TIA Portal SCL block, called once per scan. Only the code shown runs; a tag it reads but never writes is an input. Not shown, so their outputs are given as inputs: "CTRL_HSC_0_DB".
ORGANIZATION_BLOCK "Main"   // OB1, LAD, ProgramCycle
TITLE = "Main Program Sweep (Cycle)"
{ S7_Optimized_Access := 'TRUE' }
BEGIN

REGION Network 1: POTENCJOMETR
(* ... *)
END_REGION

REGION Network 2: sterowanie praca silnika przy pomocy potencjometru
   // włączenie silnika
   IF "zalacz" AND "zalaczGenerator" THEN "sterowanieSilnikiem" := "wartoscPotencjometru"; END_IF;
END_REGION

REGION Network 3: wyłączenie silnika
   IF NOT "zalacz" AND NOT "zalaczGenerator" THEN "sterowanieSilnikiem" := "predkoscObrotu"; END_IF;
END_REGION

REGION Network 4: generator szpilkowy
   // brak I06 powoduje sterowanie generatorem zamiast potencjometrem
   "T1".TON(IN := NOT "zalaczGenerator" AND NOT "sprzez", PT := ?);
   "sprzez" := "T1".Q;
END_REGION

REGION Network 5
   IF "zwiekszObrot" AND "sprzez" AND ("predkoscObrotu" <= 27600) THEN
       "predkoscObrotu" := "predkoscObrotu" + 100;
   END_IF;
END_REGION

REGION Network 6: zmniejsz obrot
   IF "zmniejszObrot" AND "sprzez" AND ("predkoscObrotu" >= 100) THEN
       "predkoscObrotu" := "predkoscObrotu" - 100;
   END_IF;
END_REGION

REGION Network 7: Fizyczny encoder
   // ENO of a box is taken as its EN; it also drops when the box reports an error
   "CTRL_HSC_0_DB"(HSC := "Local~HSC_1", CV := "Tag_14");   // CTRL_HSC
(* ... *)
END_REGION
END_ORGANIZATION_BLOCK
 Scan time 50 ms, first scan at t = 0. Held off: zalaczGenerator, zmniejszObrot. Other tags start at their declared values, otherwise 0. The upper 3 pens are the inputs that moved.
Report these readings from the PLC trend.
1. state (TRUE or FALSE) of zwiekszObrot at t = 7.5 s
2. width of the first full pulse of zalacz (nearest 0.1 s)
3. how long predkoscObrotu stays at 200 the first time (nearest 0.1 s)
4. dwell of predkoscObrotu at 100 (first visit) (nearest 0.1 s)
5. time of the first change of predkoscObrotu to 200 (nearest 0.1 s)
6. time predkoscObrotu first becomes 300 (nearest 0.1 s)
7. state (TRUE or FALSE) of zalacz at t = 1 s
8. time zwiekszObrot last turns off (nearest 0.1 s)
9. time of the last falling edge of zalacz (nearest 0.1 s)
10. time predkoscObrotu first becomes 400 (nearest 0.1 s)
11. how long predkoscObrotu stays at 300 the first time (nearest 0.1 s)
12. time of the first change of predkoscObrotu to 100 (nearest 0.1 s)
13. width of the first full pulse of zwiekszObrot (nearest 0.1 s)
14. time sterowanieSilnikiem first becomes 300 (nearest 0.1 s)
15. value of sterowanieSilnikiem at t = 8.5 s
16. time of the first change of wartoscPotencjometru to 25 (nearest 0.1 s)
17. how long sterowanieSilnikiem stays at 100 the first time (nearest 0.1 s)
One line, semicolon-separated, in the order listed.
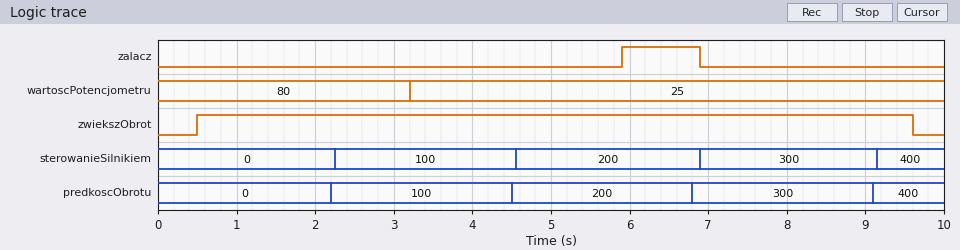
TRUE; 1.0 s; 2.3 s; 2.3 s; 4.5 s; 6.8 s; FALSE; 9.6 s; 6.9 s; 9.1 s; 2.3 s; 2.2 s; 9.1 s; 6.9 s; 300; 3.2 s; 2.3 s
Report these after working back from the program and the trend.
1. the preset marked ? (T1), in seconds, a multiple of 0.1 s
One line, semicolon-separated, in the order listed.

2.2 s
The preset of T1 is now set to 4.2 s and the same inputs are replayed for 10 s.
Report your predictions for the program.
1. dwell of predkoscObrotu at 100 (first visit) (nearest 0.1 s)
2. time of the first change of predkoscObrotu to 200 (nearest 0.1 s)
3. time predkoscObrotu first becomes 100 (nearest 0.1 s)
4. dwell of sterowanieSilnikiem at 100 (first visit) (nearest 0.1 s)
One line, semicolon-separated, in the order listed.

4.3 s; 8.5 s; 4.2 s; 4.3 s
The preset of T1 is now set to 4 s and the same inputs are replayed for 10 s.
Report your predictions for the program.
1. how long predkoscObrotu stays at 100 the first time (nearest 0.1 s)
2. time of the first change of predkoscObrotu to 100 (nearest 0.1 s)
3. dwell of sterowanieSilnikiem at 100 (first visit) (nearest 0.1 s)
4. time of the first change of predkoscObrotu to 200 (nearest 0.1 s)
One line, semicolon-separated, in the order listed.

4.1 s; 4.0 s; 4.1 s; 8.1 s
